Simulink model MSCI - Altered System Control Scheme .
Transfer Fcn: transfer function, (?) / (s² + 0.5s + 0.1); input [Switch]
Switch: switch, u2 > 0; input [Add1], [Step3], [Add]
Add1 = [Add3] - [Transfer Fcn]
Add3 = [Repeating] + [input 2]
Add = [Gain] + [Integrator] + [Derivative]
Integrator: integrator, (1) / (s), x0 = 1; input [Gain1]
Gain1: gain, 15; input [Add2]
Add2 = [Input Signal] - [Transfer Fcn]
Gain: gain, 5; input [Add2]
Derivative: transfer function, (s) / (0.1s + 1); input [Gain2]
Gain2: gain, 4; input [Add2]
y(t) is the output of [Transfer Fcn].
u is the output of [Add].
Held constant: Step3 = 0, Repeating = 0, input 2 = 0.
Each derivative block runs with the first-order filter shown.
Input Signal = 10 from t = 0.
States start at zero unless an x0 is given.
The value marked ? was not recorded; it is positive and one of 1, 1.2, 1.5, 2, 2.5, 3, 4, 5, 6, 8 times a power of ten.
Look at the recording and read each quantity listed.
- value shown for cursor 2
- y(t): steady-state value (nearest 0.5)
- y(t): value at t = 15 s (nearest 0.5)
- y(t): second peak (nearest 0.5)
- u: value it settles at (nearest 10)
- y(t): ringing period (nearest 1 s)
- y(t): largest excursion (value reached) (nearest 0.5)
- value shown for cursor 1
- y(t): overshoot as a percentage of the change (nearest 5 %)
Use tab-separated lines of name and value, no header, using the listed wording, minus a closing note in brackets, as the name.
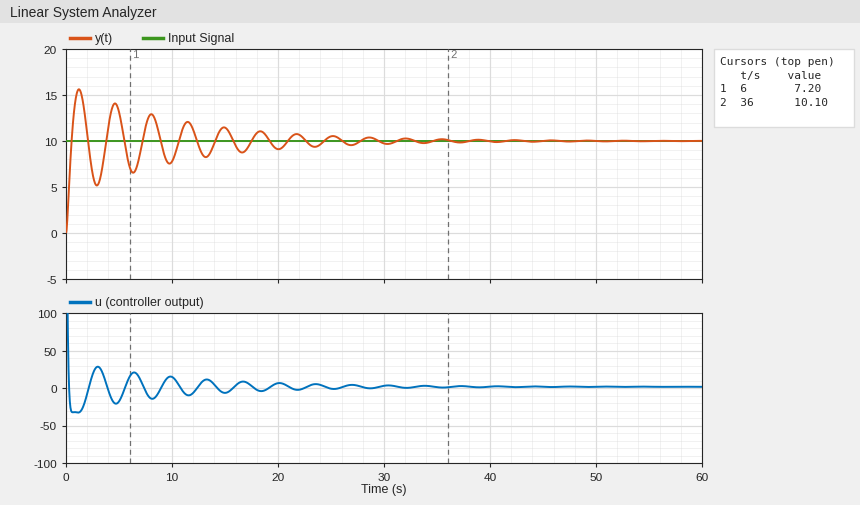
value shown for cursor 2	10.10
y(t): steady-state value	10.0
y(t): value at t = 15 s	11.5
y(t): second peak	14.0
u: value it settles at	0
y(t): ringing period	3 s
y(t): largest excursion (value reached)	15.5
value shown for cursor 1	7.20
y(t): overshoot as a percentage of the change	55 %
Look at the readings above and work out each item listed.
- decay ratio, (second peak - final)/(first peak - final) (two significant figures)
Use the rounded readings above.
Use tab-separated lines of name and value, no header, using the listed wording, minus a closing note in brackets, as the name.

decay ratio, (second peak - final)/(first peak - final)	0.73
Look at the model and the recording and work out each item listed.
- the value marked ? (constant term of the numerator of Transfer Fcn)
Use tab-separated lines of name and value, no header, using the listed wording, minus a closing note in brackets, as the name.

the value marked ?	0.6
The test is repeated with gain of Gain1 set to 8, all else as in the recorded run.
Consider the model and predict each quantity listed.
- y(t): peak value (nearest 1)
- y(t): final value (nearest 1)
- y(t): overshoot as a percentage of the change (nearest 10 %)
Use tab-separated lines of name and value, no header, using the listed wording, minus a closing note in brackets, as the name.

y(t): peak value	14
y(t): final value	10
y(t): overshoot as a percentage of the change	40 %
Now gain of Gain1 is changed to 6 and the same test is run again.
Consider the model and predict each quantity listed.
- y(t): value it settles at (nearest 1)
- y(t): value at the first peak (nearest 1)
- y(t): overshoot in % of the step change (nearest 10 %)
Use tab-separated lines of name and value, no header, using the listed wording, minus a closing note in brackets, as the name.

y(t): value it settles at	10
y(t): value at the first peak	13
y(t): overshoot in % of the step change	30 %
